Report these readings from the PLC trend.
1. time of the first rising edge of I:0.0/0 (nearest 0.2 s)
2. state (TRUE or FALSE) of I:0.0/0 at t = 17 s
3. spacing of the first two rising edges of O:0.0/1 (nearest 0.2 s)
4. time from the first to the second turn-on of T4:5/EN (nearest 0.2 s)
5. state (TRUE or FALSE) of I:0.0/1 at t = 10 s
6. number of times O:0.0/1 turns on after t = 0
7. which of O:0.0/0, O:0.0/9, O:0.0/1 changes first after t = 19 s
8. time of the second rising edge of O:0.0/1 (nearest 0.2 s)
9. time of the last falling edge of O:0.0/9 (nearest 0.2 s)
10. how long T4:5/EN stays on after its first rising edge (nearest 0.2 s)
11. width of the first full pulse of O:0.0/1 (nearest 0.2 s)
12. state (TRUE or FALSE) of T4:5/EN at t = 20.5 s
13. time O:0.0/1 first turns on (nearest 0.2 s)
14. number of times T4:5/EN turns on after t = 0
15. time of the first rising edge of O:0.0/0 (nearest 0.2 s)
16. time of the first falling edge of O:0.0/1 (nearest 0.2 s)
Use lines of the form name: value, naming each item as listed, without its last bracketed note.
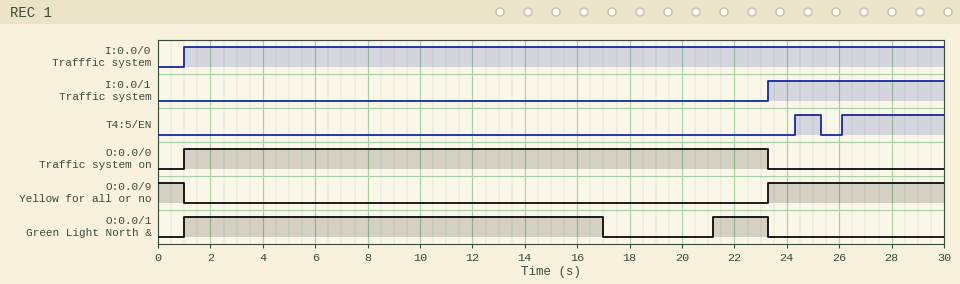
time of the first rising edge of I:0.0/0: 1.0 s
state (TRUE or FALSE) of I:0.0/0 at t = 17 s: TRUE
spacing of the first two rising edges of O:0.0/1: 20.2 s
time from the first to the second turn-on of T4:5/EN: 1.8 s
state (TRUE or FALSE) of I:0.0/1 at t = 10 s: FALSE
number of times O:0.0/1 turns on after t = 0: 2
which of O:0.0/0, O:0.0/9, O:0.0/1 changes first after t = 19 s: O:0.0/1
time of the second rising edge of O:0.0/1: 21.2 s
time of the last falling edge of O:0.0/9: 1.0 s
how long T4:5/EN stays on after its first rising edge: 1.0 s
width of the first full pulse of O:0.0/1: 16.0 s
state (TRUE or FALSE) of T4:5/EN at t = 20.5 s: FALSE
time O:0.0/1 first turns on: 1.0 s
number of times T4:5/EN turns on after t = 0: 2
time of the first rising edge of O:0.0/0: 1.0 s
time of the first falling edge of O:0.0/1: 17.0 s
